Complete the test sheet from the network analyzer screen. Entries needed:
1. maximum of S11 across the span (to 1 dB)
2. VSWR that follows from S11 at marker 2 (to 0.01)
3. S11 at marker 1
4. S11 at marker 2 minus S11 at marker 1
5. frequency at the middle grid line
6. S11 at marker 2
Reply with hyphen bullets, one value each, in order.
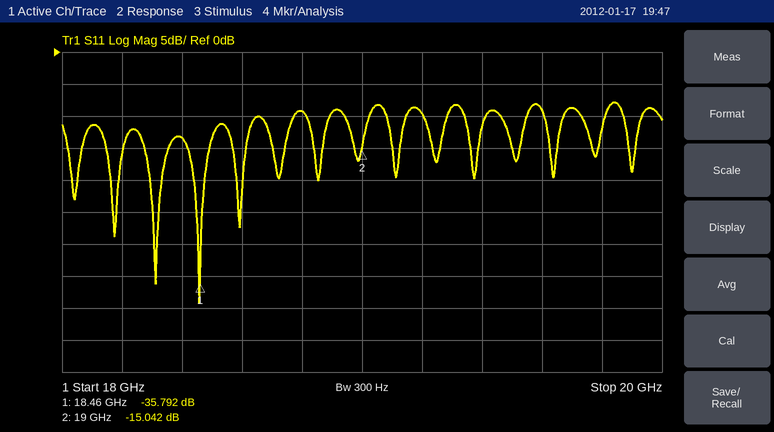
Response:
- -8 dB
- 1.43
- -35.792 dB
- 20.750 dB
- 19 GHz
- -15.042 dB
